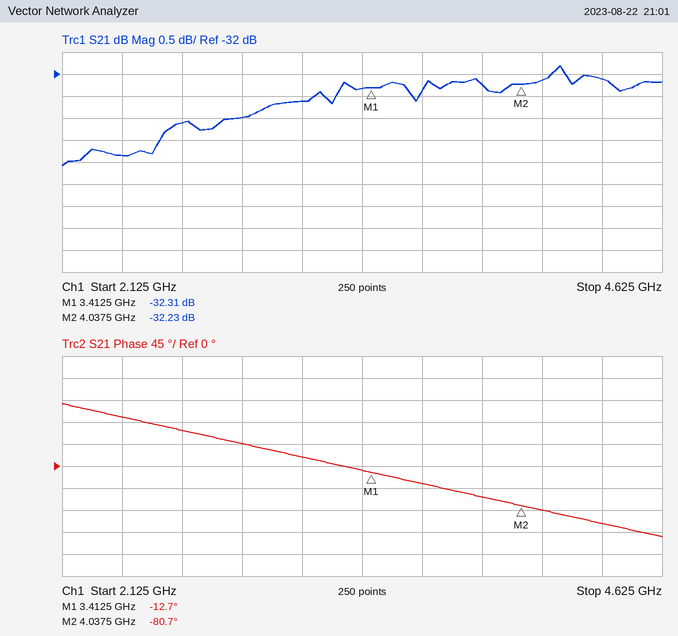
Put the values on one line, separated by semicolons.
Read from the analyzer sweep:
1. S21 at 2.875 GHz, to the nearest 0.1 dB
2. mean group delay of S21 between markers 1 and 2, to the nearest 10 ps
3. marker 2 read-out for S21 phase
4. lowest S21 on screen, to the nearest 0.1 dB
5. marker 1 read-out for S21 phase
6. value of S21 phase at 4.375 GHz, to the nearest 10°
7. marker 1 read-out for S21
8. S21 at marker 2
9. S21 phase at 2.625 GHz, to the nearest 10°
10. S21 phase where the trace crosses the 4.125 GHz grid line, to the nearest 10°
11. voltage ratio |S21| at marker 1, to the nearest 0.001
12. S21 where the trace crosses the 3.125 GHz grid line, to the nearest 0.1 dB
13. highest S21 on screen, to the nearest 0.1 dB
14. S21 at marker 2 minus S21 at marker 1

-33.0 dB; 300 ps; -80.7°; -34.1 dB; -12.7°; -120°; -32.31 dB; -32.23 dB; 70°; -90°; 0.024; -32.6 dB; -31.8 dB; 0.08 dB
